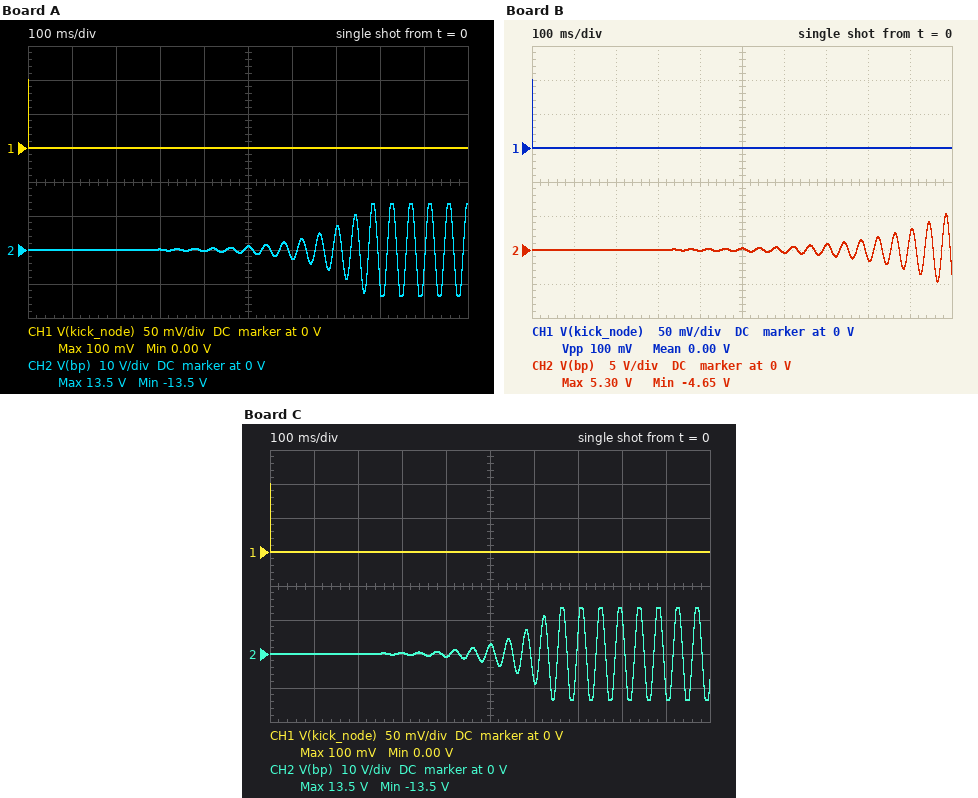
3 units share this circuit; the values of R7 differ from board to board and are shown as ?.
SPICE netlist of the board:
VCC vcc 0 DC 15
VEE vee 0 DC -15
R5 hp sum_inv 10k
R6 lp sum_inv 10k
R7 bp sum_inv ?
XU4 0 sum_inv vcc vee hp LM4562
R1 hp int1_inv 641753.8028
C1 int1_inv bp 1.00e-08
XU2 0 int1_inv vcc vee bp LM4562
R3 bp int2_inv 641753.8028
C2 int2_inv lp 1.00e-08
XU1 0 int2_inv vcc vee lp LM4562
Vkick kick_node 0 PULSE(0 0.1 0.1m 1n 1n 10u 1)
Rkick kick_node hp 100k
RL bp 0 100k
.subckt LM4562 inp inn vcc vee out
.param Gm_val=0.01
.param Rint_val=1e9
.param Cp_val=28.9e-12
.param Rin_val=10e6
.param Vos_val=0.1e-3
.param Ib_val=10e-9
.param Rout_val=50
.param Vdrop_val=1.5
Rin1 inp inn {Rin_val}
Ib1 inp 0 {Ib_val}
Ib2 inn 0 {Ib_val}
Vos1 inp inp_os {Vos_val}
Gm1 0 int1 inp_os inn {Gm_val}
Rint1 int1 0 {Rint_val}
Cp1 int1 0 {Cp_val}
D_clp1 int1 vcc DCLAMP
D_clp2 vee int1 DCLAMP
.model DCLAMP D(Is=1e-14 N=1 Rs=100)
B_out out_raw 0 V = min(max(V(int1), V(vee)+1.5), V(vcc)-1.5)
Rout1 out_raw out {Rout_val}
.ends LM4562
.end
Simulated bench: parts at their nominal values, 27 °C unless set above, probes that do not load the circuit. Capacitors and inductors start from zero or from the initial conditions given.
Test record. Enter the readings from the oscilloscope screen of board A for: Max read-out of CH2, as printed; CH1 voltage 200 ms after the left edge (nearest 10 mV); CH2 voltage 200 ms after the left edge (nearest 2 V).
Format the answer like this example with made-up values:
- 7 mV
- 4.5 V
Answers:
- 13.5 V
- 0 V
- 0 V
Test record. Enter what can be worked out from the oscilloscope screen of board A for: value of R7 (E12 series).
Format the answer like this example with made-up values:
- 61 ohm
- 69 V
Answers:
- 82 kΩ
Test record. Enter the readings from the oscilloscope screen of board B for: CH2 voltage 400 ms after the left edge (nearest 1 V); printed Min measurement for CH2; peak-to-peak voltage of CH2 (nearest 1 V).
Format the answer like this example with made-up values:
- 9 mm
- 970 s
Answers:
- 0 V
- -4.65 V
- 10 V
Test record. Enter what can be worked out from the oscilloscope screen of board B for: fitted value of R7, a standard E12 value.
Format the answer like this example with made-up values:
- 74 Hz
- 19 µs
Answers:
- 120 kΩ
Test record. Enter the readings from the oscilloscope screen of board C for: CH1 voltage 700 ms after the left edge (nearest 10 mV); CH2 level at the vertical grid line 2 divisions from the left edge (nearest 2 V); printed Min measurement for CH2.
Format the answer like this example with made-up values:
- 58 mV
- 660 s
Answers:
- 0 V
- 0 V
- -13.5 V
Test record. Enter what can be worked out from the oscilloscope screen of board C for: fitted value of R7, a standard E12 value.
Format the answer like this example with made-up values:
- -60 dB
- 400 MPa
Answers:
- 68 kΩ
